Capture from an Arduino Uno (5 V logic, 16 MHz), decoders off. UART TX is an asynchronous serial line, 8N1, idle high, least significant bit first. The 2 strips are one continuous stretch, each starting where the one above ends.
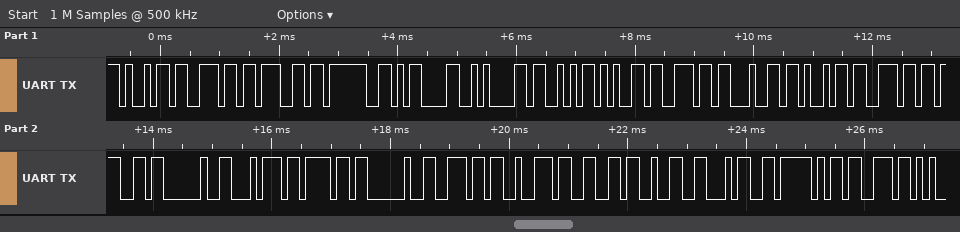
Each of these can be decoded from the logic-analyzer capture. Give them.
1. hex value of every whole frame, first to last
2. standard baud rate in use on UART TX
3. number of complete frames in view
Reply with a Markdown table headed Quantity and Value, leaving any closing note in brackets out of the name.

| Quantity | Value |
|---|---|
| hex value of every whole frame, first to last | 69 6E 67 3F 0D 0A 53 65 6E 64 69 6E 67 20 74 6F 20 6E 72 66 32 34 5F 73 |
| standard baud rate in use on UART TX | 9600 baud |
| number of complete frames in view | 24 |
